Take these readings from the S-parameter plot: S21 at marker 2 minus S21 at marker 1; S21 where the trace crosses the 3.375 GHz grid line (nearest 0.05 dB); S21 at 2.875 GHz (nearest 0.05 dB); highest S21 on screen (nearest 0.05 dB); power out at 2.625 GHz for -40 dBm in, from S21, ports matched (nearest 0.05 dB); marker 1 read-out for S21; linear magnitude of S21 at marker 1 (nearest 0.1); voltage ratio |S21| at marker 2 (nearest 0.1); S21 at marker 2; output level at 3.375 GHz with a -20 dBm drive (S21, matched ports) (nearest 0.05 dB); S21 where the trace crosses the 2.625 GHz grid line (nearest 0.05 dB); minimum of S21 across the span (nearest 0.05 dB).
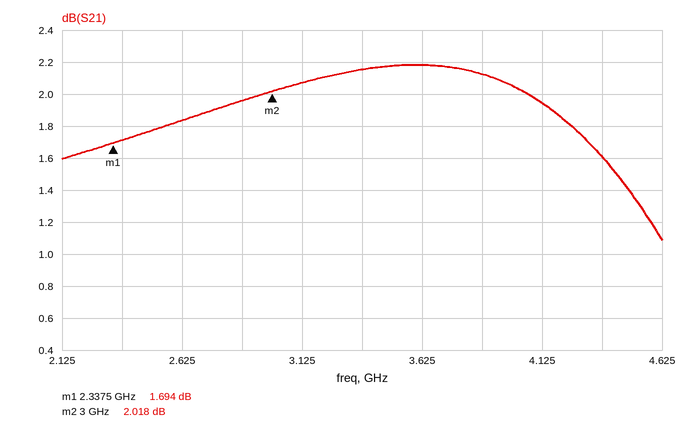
0.324 dB
2.15 dB
1.95 dB
2.20 dB
-38.15 dBm
1.694 dB
1.2
1.3
2.018 dB
-17.85 dBm
1.85 dB
1.10 dB
